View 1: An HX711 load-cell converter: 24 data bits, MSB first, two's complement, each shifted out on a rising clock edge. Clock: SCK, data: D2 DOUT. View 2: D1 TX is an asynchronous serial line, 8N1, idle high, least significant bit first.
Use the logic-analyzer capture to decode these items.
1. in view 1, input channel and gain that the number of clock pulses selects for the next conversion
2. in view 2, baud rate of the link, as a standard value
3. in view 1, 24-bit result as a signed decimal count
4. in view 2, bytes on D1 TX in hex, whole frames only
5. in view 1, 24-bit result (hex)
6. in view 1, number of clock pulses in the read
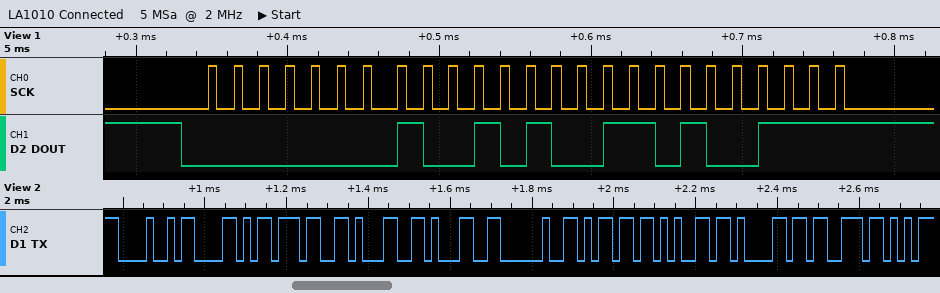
channel A, gain 128
57600 baud
76199
48 58 37 31 31 20 6D 65 61 73
0x0129A7
25
